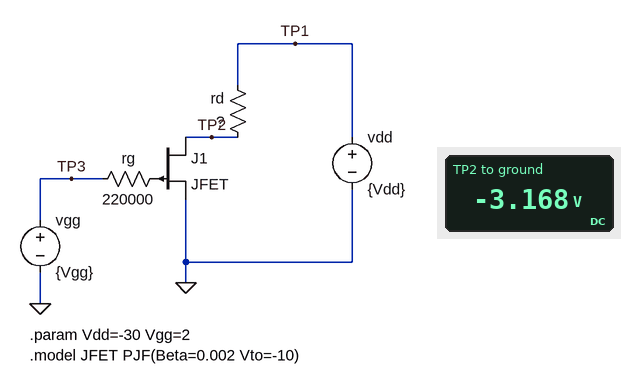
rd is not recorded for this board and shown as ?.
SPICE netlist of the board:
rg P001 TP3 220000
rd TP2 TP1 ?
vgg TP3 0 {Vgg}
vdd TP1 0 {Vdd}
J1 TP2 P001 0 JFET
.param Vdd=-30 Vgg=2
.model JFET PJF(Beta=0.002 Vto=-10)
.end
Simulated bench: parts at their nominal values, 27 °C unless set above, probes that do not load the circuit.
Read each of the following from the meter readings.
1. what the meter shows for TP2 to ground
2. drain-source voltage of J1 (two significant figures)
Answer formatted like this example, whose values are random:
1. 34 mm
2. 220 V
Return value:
1. -3.168 V
2. -3.2 V
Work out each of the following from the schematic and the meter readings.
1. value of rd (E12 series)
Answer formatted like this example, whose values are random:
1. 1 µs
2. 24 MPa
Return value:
1. 330 Ω
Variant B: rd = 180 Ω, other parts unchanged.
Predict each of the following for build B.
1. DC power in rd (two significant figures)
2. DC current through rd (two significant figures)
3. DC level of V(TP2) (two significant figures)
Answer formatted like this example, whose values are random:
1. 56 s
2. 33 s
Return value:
1. 2.9 W
2. 130 mA
3. -7.2 V
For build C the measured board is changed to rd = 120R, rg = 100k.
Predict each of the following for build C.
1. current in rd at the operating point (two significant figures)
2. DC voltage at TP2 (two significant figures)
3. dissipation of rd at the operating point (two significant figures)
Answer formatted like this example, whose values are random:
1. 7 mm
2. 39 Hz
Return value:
1. 130 mA
2. -15 V
3. 2.0 W
